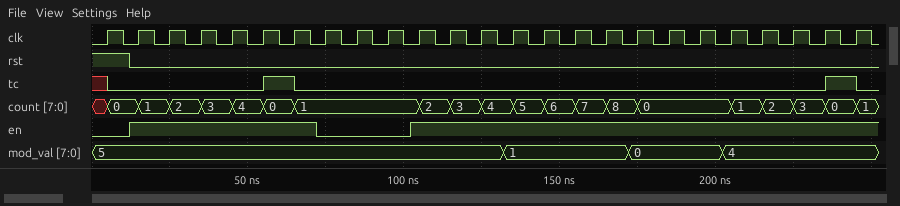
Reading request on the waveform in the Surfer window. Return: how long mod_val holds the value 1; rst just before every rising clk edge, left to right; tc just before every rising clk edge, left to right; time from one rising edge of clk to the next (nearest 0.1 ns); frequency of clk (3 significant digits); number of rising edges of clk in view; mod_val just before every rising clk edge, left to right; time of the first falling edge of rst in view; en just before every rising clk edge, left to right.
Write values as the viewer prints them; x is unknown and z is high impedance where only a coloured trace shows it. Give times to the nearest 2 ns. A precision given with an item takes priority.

40 ns
1 0 0 0 0 0 0 0 0 0 0 0 0 0 0 0 0 0 0 0 0 0 0 0 0
x 0 0 0 0 0 1 0 0 0 0 0 0 0 0 0 0 0 0 0 0 0 0 0 1
10 ns
100 MHz
25
5, 5, 5, 5, 5, 5, 5, 5, 5, 5, 5, 5, 5, 1, 1, 1, 1, 0, 0, 0, 4, 4, 4, 4, 4
12 ns
0 1 1 1 1 1 1 0 0 0 1 1 1 1 1 1 1 1 1 1 1 1 1 1 1
